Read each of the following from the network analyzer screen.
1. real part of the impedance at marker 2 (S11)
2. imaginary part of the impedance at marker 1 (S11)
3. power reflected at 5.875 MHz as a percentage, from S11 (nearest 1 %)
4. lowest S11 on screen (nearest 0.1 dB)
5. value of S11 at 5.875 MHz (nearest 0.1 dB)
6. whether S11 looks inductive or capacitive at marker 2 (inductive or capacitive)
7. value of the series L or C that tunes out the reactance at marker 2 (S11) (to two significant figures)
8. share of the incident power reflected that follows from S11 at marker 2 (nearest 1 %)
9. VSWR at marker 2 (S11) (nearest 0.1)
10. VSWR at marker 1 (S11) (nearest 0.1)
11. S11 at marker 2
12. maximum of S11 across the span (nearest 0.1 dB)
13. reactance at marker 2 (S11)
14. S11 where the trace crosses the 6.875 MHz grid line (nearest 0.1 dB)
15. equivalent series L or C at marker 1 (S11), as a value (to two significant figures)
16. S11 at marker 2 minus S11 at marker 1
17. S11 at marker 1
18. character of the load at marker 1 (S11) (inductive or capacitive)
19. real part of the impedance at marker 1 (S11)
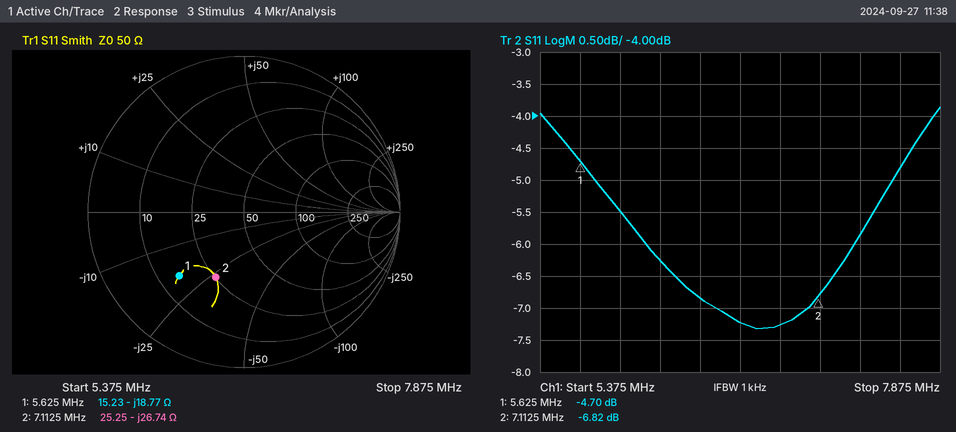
25.25 Ω
-18.77 Ω
28 %
-7.3 dB
-5.5 dB
capacitive
600 nH
21 %
2.7
3.8
-6.82 dB
-3.9 dB
-26.74 Ω
-7.3 dB
1.5 nF
-2.12 dB
-4.70 dB
capacitive
15.23 Ω
